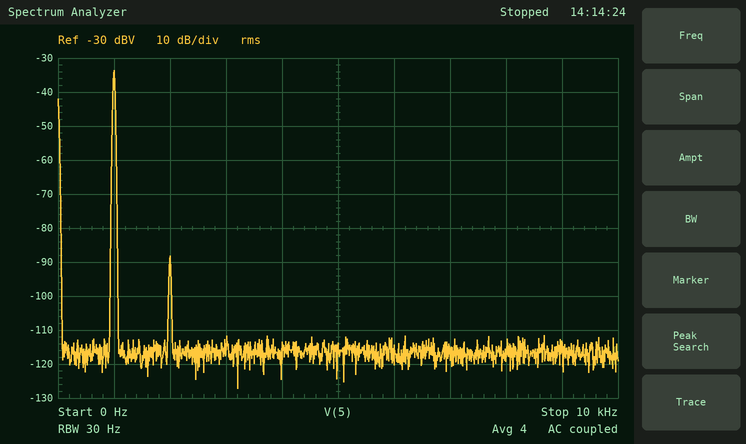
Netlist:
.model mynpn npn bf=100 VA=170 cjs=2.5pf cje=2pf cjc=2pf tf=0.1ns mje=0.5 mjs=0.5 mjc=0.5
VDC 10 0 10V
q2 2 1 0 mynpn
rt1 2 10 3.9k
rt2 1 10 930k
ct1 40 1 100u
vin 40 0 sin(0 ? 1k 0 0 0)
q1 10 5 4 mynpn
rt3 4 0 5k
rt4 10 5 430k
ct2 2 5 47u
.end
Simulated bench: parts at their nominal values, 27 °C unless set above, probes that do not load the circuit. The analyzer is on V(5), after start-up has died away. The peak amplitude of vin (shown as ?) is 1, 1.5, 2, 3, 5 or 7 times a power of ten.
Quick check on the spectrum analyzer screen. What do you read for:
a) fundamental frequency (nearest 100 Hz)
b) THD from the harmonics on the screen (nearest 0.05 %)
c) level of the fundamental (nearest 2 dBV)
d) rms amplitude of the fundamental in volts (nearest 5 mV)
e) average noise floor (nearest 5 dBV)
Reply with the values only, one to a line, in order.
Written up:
1.0 kHz
0.20 %
-34 dBV
20 mV
-115 dBV
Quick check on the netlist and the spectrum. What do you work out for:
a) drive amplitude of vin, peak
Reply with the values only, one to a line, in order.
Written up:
200 µV
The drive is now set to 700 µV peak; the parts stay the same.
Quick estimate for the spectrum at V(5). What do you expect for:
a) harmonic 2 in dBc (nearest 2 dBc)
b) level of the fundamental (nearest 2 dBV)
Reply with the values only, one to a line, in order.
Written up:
-44 dBc
-22 dBV
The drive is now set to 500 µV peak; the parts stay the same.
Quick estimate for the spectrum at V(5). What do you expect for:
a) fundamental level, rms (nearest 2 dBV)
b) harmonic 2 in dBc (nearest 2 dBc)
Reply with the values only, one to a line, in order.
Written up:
-26 dBV
-46 dBc
